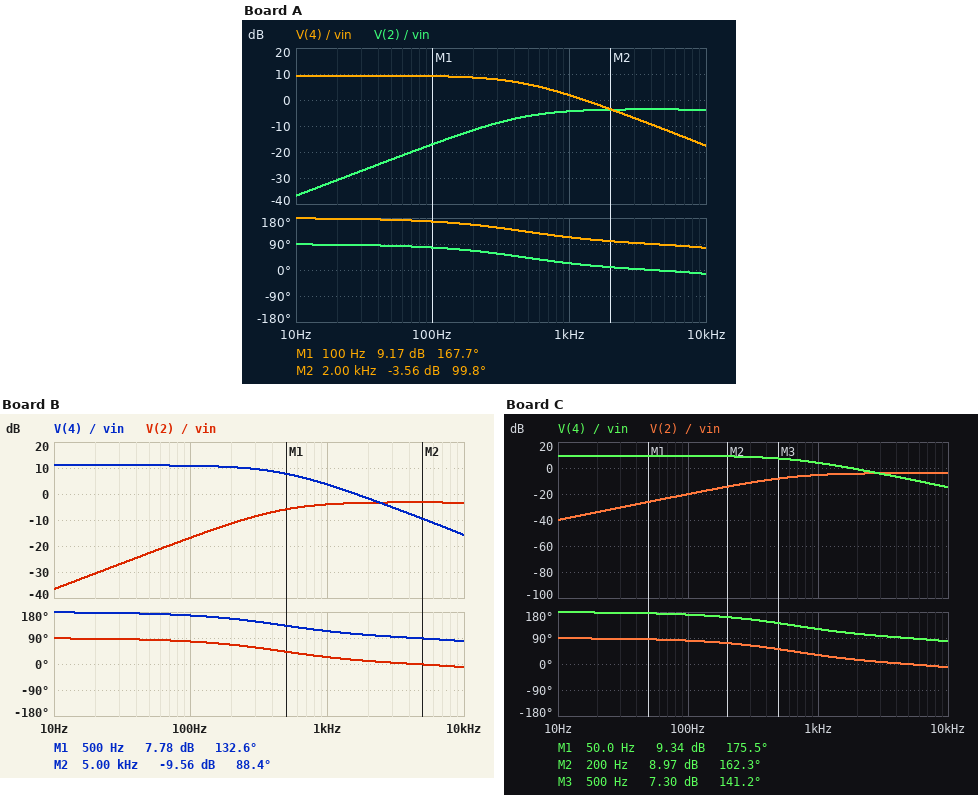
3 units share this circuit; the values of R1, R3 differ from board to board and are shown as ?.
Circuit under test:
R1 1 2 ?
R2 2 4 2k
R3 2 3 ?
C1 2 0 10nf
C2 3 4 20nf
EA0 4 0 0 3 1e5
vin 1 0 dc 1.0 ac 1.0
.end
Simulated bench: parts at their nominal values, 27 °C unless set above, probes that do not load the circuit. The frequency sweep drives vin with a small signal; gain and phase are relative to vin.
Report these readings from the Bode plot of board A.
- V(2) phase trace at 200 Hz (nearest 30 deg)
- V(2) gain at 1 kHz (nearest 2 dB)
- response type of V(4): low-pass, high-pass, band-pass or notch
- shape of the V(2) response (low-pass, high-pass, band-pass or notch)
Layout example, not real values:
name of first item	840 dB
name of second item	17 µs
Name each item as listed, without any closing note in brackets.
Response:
V(2) phase trace at 200 Hz	60 deg
V(2) gain at 1 kHz	-4 dB
response type of V(4): low-pass, high-pass, band-pass or notch	low-pass
shape of the V(2) response	high-pass
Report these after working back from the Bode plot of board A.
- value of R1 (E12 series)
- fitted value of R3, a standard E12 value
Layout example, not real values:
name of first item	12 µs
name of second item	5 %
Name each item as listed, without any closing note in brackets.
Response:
value of R1	680 Ω
fitted value of R3, a standard E12 value	3.9 kΩ
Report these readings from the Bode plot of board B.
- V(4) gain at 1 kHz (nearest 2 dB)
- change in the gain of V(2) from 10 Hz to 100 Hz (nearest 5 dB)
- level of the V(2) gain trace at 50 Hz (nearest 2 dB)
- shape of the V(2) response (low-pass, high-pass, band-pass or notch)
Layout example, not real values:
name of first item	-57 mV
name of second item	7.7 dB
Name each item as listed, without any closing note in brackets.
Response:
V(4) gain at 1 kHz	4 dB
change in the gain of V(2) from 10 Hz to 100 Hz	20 dB
level of the V(2) gain trace at 50 Hz	-22 dB
shape of the V(2) response	high-pass
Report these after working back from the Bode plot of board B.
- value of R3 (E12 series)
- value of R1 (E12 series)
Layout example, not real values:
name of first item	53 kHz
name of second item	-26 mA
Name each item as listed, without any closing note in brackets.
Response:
value of R3	3.3 kΩ
value of R1	560 Ω
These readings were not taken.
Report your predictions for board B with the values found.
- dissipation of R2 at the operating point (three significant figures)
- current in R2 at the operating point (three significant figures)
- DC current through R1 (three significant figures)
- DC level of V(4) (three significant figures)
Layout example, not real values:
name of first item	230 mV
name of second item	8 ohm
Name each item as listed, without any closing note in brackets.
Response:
dissipation of R2 at the operating point	6.38 mW
current in R2 at the operating point	1.79 mA
DC current through R1	1.79 mA
DC level of V(4)	-3.57 V
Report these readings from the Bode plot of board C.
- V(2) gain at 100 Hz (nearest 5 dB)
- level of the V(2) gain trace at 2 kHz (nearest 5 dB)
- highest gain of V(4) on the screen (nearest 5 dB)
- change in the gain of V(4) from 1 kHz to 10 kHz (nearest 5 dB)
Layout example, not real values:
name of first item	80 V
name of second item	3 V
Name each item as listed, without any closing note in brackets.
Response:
V(2) gain at 100 Hz	-20 dB
level of the V(2) gain trace at 2 kHz	-5 dB
highest gain of V(4) on the screen	10 dB
change in the gain of V(4) from 1 kHz to 10 kHz	-20 dB
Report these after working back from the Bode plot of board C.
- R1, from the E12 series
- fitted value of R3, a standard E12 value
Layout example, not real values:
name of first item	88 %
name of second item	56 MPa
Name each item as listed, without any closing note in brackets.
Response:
R1, from the E12 series	680 Ω
fitted value of R3, a standard E12 value	2.7 kΩ
